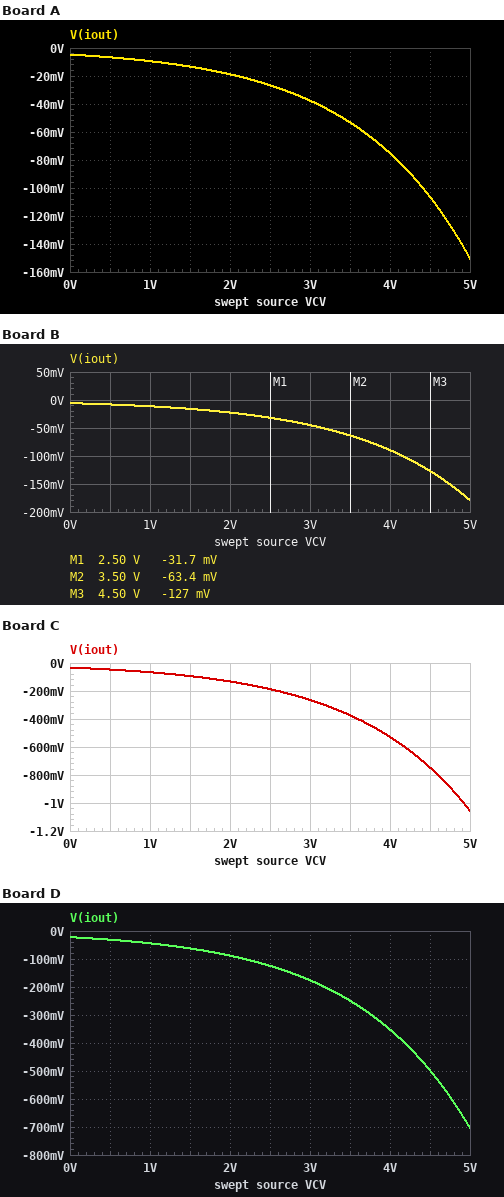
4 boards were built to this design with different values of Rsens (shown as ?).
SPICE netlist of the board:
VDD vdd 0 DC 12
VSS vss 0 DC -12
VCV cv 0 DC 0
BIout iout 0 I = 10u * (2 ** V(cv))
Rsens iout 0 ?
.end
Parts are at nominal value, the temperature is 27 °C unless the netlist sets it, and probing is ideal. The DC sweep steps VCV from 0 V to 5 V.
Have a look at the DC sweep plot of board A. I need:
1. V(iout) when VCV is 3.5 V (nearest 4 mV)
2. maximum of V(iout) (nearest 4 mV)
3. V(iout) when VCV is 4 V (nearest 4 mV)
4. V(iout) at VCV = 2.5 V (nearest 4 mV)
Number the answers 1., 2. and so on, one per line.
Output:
1. -52 mV
2. -4 mV
3. -76 mV
4. -28 mV
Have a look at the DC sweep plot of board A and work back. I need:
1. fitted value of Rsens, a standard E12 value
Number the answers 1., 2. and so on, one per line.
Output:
1. 470 Ω
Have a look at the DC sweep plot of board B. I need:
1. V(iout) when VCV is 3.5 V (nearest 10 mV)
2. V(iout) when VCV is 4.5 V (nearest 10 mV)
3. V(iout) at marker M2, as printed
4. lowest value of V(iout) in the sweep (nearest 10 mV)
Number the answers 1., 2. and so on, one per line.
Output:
1. -60 mV
2. -130 mV
3. -63.4 mV
4. -180 mV
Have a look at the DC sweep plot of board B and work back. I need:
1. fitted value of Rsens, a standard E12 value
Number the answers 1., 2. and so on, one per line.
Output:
1. 560 Ω
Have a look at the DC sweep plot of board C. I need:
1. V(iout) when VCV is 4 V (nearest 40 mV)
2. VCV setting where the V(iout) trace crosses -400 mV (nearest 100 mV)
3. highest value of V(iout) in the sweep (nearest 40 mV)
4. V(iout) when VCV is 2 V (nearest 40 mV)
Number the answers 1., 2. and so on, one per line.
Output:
1. -520 mV
2. 3.6 V
3. -40 mV
4. -120 mV
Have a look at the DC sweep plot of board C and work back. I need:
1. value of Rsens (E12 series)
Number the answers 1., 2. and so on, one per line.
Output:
1. 3.3 kΩ
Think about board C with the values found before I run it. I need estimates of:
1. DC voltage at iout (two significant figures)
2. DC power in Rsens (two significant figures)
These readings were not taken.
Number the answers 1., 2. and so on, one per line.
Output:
1. -33 mV
2. 330 nW
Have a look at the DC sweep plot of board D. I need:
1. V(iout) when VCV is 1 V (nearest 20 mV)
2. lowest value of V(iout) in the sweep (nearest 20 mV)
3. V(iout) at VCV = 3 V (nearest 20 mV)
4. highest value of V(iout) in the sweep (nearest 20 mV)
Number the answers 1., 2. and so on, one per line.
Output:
1. -40 mV
2. -700 mV
3. -180 mV
4. -20 mV
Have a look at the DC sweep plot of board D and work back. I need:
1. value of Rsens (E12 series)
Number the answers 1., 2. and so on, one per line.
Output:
1. 2.2 kΩ
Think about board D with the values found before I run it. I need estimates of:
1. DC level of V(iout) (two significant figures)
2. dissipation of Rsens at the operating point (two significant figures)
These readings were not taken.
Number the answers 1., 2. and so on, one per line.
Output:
1. -22 mV
2. 220 nW
